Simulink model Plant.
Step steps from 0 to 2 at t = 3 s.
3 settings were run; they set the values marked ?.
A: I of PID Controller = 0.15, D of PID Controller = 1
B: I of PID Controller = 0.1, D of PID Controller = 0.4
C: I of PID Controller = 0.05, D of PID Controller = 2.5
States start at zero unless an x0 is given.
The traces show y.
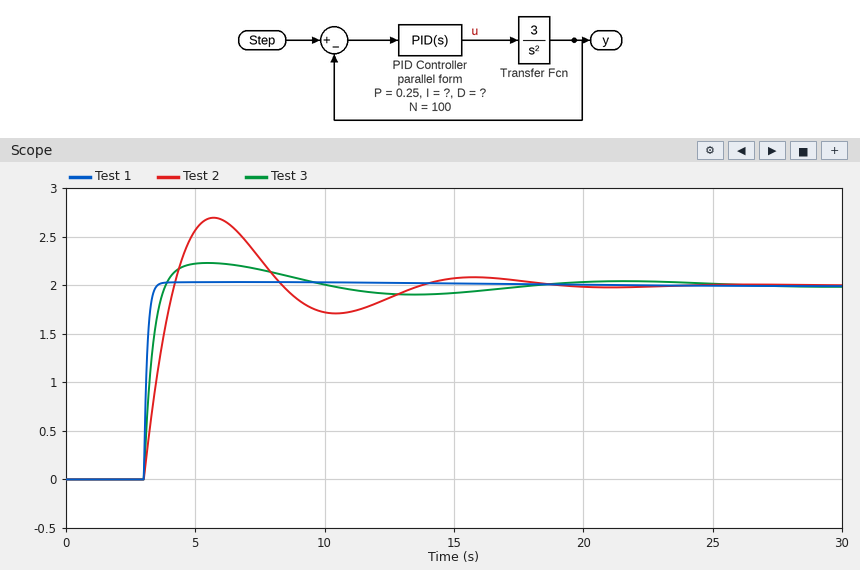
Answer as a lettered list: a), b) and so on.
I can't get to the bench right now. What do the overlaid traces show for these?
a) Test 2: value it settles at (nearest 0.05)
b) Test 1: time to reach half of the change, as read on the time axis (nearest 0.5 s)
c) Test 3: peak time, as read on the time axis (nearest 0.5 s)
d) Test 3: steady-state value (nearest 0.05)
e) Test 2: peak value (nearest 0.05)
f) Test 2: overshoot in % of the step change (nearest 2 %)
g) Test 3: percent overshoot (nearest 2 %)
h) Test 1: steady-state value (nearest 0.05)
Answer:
a) 2.00
b) 3.0 s
c) 5.5 s
d) 2.00
e) 2.70
f) 34 %
g) 12 %
h) 2.00
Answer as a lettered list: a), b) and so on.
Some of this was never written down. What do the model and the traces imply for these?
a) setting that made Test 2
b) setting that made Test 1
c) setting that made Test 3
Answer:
a) B
b) C
c) A
